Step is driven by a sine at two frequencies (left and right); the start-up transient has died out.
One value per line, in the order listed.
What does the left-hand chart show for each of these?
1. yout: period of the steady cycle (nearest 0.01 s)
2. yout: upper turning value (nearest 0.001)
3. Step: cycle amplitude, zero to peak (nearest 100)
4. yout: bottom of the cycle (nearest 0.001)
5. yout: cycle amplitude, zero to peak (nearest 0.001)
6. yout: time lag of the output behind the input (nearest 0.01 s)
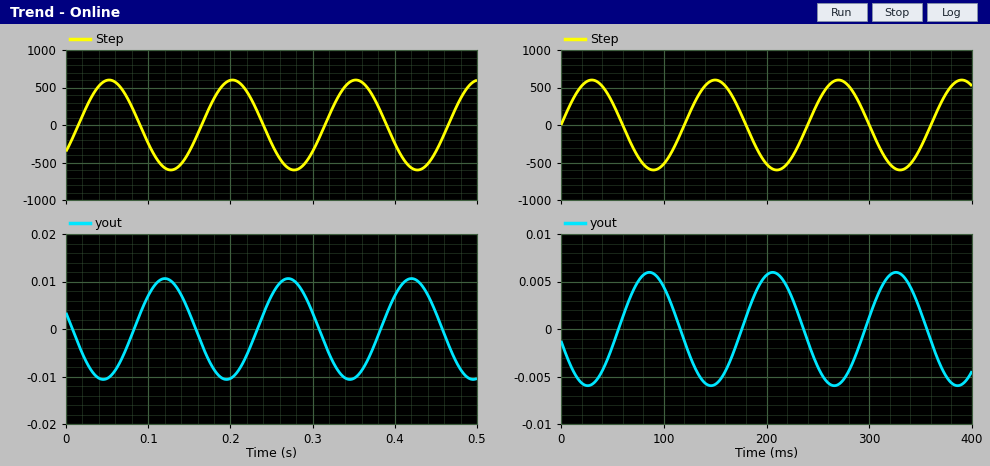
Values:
0.15 s
0.011
600
-0.011
0.011
0.07 s
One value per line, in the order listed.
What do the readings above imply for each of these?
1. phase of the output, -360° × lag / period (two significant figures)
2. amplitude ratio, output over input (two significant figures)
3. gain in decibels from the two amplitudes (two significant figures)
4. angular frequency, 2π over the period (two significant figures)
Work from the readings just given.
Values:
-170°
0.000018
-95 dB
42 rad/s
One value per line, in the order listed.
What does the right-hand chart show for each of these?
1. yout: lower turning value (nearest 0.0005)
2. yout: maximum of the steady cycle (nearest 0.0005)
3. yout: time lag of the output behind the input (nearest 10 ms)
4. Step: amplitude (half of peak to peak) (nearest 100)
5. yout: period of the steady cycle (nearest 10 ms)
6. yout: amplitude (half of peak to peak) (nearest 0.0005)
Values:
-0.0060
0.0060
60 ms
600
120 ms
0.0060
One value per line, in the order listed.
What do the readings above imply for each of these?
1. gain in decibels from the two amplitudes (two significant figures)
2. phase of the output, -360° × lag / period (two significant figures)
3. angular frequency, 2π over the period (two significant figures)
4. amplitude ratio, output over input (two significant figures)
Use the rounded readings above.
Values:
-100 dB
-180°
0.052 rad/ms
0.000010
